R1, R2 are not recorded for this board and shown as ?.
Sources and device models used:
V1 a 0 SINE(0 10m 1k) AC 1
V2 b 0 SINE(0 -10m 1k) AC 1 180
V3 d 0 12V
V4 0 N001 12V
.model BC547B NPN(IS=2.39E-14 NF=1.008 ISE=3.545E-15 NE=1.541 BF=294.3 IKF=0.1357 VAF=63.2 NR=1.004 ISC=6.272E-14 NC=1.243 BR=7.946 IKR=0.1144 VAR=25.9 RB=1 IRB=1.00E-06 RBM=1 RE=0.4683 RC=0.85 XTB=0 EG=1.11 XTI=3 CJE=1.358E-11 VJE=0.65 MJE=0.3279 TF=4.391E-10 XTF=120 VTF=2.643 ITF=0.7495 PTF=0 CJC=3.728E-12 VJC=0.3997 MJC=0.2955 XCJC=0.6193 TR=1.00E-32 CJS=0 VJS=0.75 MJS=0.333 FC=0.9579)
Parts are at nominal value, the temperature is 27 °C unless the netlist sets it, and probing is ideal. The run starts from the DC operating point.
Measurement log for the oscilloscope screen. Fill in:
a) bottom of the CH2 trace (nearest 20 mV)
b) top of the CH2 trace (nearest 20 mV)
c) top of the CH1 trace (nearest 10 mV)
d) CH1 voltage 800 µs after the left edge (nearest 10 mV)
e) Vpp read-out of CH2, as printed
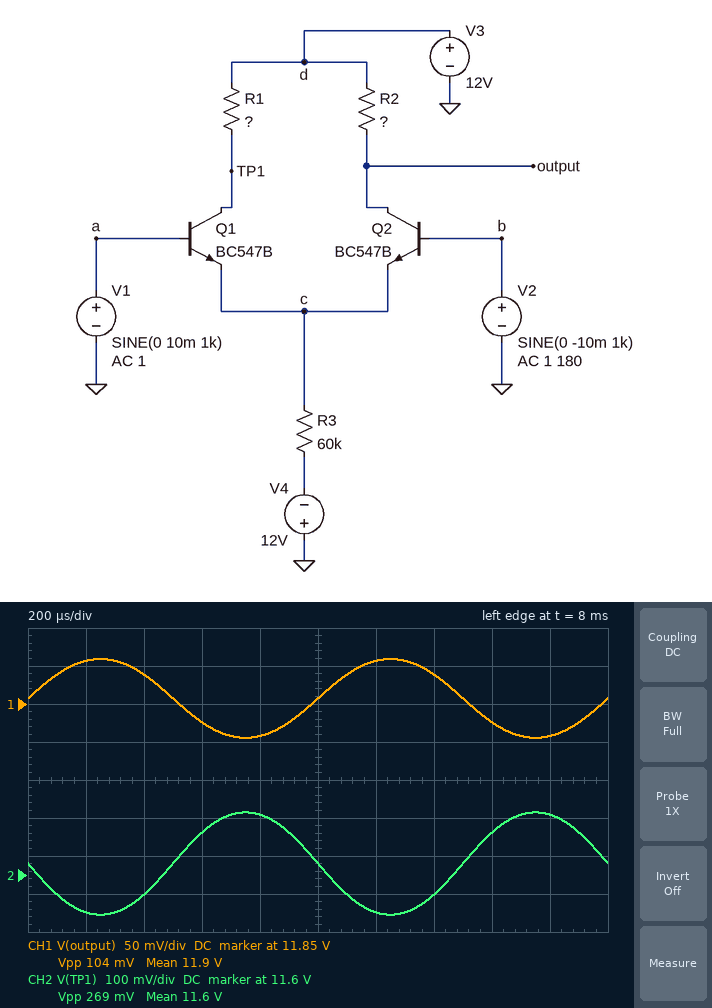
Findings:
11.50 V
11.76 V
11.91 V
11.81 V
269 mV
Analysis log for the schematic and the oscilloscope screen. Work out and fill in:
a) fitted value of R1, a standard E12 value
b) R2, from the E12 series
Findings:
3.9 kΩ
1.5 kΩ
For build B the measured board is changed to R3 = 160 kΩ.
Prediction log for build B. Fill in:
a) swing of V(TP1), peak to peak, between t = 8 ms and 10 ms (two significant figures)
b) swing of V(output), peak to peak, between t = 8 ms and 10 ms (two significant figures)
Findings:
100 mV
39 mV
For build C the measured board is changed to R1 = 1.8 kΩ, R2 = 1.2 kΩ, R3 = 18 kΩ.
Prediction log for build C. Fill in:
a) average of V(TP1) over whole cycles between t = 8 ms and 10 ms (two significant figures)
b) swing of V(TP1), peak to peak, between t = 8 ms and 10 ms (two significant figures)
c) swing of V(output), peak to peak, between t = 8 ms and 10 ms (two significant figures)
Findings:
11 V
410 mV
270 mV
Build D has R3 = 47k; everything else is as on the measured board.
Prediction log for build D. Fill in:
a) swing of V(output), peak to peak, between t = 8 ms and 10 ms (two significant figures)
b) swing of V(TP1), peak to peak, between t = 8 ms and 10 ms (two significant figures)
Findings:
130 mV
340 mV
